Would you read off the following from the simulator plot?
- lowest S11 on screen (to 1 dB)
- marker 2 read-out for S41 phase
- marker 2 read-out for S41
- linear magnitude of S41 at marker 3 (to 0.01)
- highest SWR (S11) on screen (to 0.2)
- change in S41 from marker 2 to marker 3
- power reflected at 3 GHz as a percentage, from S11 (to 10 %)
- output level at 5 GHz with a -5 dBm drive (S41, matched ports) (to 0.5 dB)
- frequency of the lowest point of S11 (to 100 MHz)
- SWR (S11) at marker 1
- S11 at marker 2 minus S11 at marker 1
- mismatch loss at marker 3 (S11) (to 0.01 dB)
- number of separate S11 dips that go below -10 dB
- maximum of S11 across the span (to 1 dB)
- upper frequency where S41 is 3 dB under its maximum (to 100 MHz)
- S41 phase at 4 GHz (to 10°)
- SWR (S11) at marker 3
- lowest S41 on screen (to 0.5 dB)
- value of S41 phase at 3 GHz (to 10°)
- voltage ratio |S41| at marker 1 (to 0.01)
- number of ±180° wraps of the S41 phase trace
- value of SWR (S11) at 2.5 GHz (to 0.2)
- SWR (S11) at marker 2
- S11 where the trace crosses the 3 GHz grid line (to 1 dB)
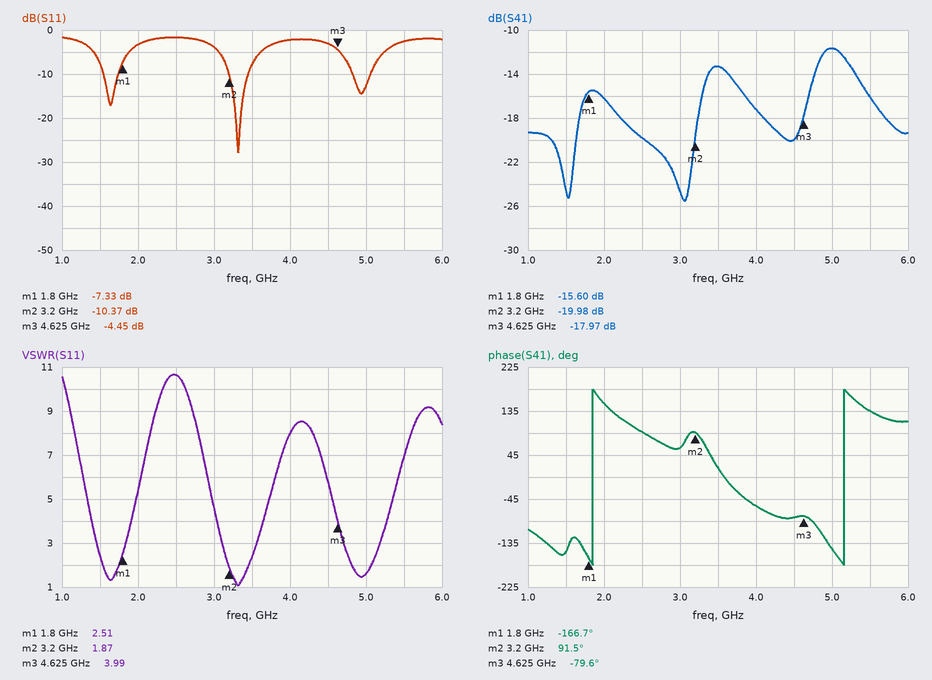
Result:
-28 dB
91.5°
-19.98 dB
0.13
10.6
2.01 dB
40 %
-16.5 dBm
3.3 GHz
2.51
-3.04 dB
1.93 dB
3
-2 dB
5.4 GHz
-60°
3.99
-25.5 dB
60°
0.17
2
10.6
1.87
-4 dB
